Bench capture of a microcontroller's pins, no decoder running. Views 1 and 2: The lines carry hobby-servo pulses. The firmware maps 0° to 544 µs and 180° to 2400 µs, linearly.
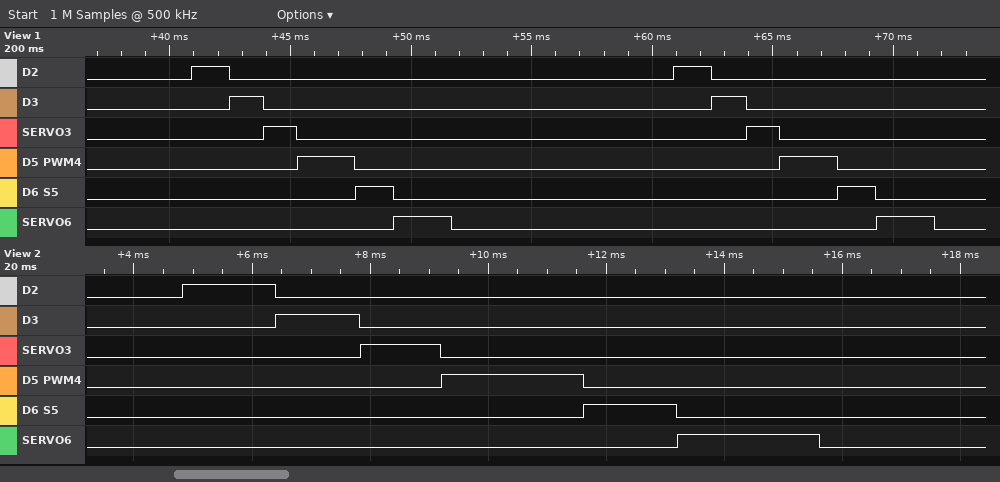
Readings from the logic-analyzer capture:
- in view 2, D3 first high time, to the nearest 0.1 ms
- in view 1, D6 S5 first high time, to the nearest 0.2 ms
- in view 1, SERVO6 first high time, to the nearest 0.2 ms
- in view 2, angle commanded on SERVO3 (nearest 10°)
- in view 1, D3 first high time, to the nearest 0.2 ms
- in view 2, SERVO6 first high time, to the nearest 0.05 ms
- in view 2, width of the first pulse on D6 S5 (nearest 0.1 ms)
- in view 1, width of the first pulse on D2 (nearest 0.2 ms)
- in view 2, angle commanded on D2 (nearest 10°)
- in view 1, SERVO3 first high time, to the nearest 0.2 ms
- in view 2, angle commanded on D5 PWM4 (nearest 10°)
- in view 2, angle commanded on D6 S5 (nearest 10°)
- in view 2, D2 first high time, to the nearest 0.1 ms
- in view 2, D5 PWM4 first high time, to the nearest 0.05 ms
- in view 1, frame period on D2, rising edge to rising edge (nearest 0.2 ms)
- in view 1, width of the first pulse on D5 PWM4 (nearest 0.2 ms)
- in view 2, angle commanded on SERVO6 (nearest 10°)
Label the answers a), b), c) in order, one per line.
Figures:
a) 1.4 ms
b) 1.6 ms
c) 2.4 ms
d) 80°
e) 1.4 ms
f) 2.40 ms
g) 1.6 ms
h) 1.6 ms
i) 100°
j) 1.4 ms
k) 180°
l) 100°
m) 1.6 ms
n) 2.40 ms
o) 20.0 ms
p) 2.4 ms
q) 180°
